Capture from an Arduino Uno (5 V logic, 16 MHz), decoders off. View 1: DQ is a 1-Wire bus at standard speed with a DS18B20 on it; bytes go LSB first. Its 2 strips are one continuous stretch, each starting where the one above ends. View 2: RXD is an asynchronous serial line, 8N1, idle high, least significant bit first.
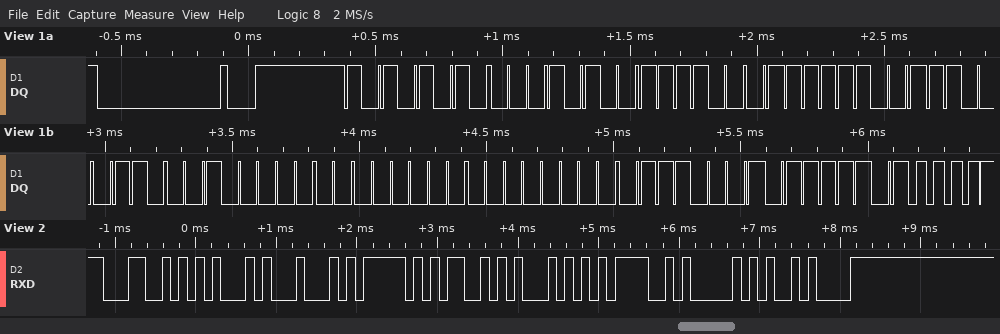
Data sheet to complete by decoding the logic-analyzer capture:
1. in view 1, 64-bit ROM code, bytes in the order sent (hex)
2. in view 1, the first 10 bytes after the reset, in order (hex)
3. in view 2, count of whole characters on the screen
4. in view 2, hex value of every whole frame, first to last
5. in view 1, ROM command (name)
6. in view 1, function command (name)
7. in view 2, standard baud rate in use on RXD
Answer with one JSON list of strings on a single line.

["28 8F 9F 63 04 00 00 8E", "55 28 8F 9F 63 04 00 00 8E BE", "9", "4C 45 44 5F 53 54 4F 50 0A", "Match ROM", "Read Scratchpad", "9600 baud"]
